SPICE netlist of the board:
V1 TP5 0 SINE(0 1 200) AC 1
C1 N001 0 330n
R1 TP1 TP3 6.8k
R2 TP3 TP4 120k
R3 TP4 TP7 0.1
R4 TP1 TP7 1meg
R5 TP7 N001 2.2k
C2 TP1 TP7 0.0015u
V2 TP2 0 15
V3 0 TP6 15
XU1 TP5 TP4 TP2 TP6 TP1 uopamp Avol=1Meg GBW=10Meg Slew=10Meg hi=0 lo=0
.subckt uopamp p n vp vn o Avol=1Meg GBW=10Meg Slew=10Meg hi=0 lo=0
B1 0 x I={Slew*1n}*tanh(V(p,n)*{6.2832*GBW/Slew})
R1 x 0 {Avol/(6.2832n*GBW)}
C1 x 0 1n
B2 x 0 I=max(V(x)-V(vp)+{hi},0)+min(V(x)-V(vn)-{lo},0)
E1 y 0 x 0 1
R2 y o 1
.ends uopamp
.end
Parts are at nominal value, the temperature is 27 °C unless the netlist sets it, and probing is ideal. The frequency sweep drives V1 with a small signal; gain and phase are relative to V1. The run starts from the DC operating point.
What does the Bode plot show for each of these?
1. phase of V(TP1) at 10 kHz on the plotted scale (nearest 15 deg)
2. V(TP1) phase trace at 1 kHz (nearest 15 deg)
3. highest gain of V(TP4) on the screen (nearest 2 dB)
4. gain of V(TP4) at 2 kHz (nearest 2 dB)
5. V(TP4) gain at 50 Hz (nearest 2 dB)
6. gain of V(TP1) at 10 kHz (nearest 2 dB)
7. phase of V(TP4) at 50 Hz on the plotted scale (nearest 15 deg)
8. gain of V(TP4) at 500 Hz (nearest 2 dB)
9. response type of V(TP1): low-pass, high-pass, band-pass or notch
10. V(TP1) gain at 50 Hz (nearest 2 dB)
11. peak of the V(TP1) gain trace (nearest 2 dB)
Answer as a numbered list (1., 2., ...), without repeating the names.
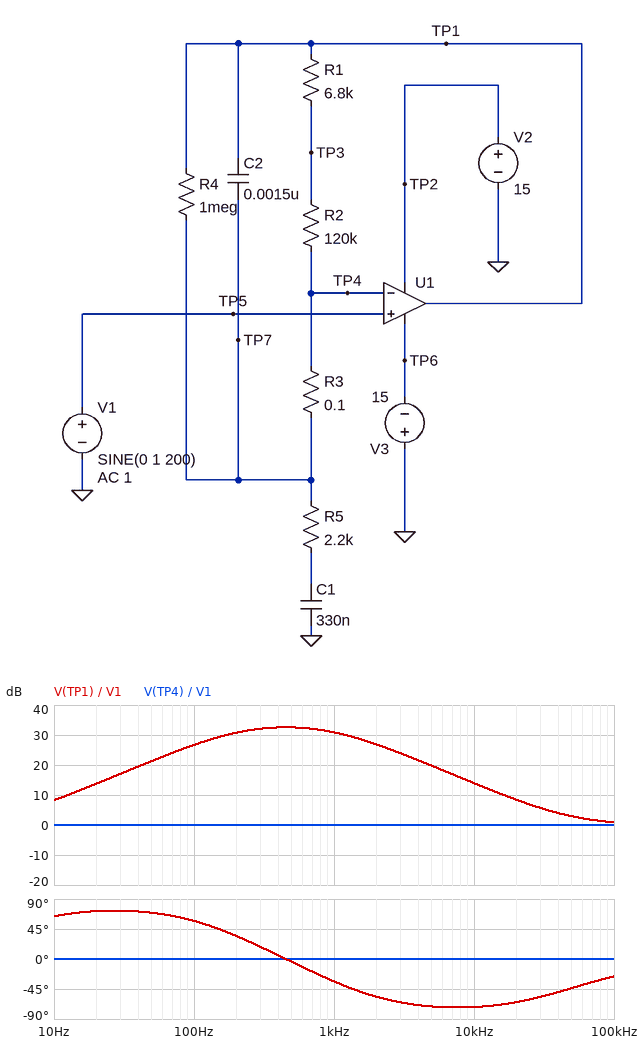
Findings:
1. -75 deg
2. -30 deg
3. 0 dB
4. 0 dB
5. 0 dB
6. 14 dB
7. 0 deg
8. 0 dB
9. band-pass
10. 22 dB
11. 32 dB
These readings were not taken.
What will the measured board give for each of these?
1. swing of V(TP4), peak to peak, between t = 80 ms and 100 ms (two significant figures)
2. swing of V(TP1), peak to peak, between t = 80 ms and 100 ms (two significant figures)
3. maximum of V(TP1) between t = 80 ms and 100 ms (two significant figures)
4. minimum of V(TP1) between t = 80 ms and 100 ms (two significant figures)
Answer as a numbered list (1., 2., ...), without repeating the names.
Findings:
1. 1.4 V
2. 30 V
3. 15 V
4. -15 V
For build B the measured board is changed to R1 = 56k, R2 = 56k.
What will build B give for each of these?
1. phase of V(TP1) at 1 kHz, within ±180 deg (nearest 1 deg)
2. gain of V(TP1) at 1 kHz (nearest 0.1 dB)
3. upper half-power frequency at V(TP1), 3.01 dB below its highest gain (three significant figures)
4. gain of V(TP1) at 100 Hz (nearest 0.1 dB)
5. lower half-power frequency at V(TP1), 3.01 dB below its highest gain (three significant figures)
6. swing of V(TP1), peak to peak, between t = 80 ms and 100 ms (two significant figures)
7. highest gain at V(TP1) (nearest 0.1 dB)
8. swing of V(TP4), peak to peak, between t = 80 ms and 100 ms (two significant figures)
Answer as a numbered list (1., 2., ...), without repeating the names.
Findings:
1. -30 deg
2. 30.4 dB
3. 1.43 kHz
4. 25.8 dB
5. 161 Hz
6. 30 V
7. 31.8 dB
8. 1.5 V
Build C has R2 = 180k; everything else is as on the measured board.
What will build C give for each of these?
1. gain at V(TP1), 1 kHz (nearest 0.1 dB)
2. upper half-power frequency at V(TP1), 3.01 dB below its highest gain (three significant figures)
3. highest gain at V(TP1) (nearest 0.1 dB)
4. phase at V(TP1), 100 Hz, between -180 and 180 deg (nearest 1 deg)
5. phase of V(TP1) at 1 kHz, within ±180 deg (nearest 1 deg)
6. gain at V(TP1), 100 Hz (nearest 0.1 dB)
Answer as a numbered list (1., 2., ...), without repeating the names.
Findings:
1. 32.0 dB
2. 1.03 kHz
3. 34.8 dB
4. 55 deg
5. -43 deg
6. 29.5 dB
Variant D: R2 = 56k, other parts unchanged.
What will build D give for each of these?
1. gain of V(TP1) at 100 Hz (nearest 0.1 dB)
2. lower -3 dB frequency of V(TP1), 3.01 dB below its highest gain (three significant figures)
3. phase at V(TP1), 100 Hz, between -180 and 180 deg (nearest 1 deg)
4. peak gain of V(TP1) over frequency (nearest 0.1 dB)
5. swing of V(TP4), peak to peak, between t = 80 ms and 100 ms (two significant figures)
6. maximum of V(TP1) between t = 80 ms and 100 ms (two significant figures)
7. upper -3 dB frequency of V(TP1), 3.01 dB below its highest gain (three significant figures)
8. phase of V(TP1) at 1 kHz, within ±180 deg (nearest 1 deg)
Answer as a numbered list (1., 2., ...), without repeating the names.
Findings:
1. 21.3 dB
2. 179 Hz
3. 58 deg
4. 27.9 dB
5. 2.0 V
6. 15 V
7. 2.19 kHz
8. -16 deg
